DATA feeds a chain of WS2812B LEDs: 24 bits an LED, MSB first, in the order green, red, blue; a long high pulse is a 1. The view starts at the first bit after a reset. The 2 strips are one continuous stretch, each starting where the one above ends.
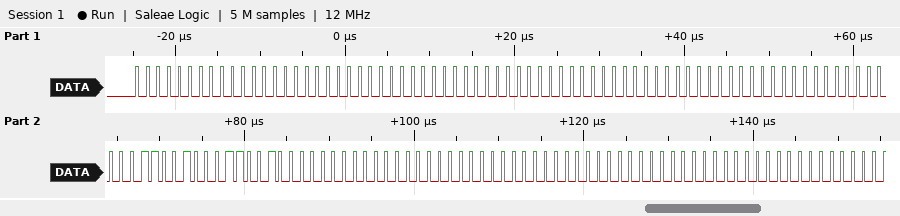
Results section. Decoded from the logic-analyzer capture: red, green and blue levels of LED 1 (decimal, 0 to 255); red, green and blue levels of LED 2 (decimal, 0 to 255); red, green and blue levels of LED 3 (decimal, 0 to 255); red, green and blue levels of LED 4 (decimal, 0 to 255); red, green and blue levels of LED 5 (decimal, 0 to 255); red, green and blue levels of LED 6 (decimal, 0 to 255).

0, 0, 0
0, 0, 0
0, 0, 0
50, 50, 0
0, 0, 0
0, 0, 0
